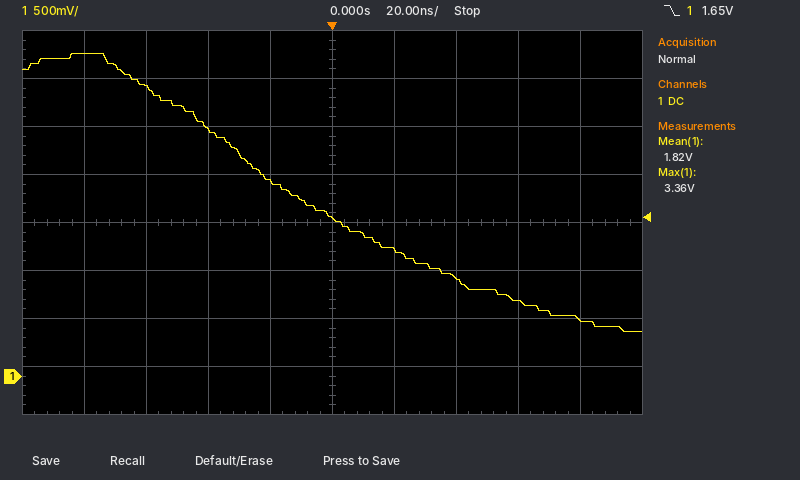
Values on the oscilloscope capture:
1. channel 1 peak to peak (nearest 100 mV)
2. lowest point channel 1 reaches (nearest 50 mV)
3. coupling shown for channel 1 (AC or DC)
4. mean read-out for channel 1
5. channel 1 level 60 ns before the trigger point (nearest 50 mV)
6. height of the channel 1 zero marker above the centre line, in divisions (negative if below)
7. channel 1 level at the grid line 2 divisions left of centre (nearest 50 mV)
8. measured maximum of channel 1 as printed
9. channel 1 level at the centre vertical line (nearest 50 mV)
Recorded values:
2.90 V
450 mV
DC
1.82 V
3.00 V
-3.2 div
2.55 V
3.36 V
1.65 V
